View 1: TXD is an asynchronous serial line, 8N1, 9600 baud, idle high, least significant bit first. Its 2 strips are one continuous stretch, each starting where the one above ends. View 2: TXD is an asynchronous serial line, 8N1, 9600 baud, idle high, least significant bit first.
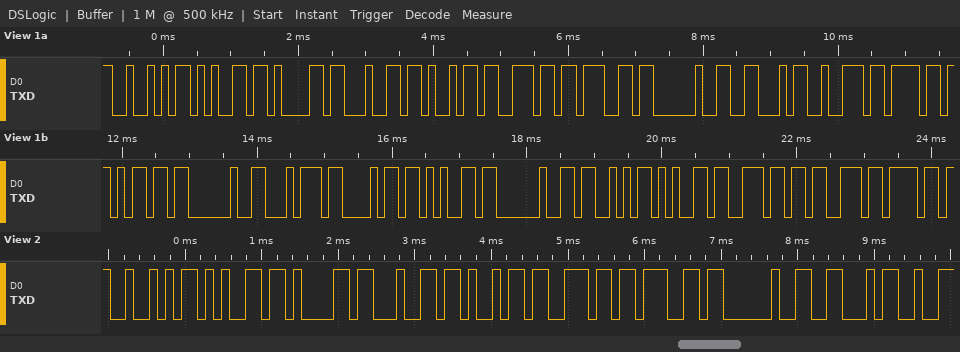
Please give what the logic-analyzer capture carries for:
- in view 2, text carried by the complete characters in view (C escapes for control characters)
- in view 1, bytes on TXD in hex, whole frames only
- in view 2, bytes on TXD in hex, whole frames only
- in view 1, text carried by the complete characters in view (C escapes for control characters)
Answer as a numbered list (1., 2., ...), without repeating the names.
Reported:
1. "Reading F"
2. 0x52 0x65 0x61 0x64 0x69 0x6E 0x67 0x20 0x46 0x72 0x6F 0x6D 0x20 0x74 0x68 0x65 0x20 0x53 0x65 0x6E 0x73 0x6F
3. 52 65 61 64 69 6E 67 20 46
4. "Reading From the Senso"
